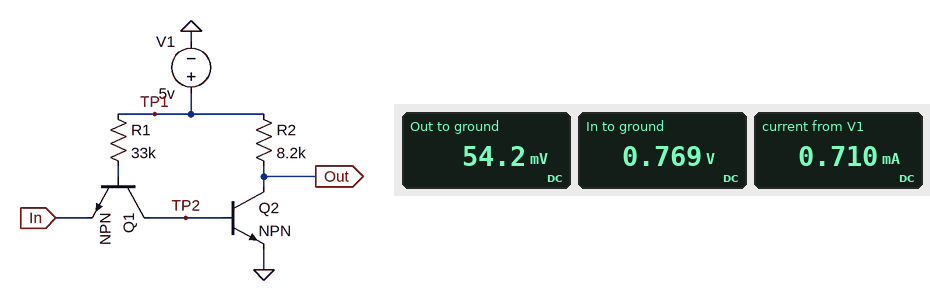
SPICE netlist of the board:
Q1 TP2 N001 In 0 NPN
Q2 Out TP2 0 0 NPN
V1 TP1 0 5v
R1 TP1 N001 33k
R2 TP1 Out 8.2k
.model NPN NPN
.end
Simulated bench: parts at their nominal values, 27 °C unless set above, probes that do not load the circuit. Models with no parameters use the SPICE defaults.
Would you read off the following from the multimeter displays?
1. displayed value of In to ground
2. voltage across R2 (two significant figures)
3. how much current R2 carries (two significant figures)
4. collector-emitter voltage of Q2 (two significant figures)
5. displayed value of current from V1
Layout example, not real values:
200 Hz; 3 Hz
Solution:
0.769 V; 4.9 V; 600 µA; 54 mV; 0.710 mA
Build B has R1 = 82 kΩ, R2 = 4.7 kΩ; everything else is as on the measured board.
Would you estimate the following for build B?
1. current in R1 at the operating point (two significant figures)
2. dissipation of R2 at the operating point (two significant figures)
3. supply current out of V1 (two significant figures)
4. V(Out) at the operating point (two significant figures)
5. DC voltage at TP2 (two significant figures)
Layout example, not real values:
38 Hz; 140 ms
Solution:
43 µA; 5.1 mW; 1.1 mA; 92 mV; 780 mV
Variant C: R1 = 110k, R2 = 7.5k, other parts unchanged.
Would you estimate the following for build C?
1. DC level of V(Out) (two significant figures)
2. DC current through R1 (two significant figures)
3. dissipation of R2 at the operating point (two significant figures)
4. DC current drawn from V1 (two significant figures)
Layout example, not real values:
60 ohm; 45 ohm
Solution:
86 mV; 32 µA; 3.2 mW; 690 µA
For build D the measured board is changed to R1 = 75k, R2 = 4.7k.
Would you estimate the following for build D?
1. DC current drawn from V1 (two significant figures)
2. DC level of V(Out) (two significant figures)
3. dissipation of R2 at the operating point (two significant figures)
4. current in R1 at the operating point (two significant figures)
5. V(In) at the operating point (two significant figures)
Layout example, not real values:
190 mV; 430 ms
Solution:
1.1 mA; 89 mV; 5.1 mW; 47 µA; 780 mV
